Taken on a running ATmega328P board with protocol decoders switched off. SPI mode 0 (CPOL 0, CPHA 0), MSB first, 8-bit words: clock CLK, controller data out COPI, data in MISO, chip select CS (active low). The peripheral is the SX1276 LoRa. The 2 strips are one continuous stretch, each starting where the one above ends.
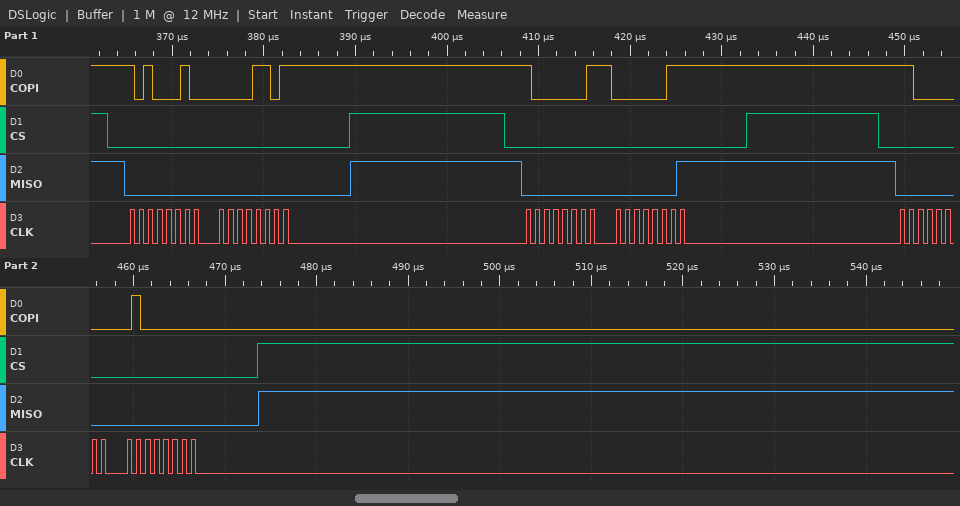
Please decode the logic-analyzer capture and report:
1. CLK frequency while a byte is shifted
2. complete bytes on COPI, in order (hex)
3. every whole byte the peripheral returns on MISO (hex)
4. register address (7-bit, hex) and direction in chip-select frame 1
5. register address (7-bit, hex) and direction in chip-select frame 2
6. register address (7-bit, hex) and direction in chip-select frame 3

1 MHz
A2 0D 81 03 C0 40
00 00 00 01 00 00
0x22 write
0x01 write
0x40 write
